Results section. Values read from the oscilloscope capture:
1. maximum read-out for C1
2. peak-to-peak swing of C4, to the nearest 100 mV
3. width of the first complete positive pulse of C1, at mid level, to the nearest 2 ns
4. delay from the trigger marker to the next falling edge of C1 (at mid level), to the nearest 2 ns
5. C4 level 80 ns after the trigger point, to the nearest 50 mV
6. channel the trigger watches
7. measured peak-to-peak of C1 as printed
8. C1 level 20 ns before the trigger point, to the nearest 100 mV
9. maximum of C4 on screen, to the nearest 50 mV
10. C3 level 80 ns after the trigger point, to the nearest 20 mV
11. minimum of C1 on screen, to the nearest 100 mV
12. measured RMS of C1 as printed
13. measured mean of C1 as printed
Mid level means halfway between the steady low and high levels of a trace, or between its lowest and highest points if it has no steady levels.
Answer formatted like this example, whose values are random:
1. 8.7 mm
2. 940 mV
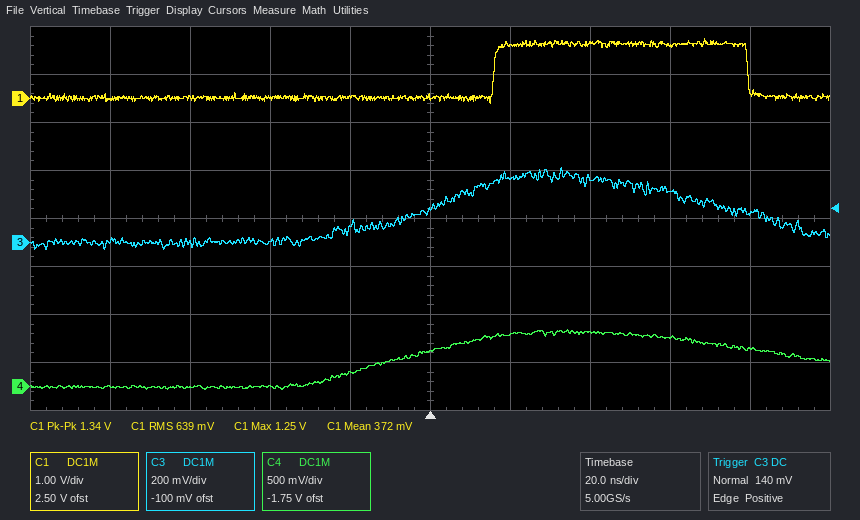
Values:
1. 1.25 V
2. 600 mV
3. 64 ns
4. 80 ns
5. 400 mV
6. C3
7. 1.34 V
8. 0.0 V
9. 600 mV
10. 120 mV
11. -100 mV
12. 639 mV
13. 372 mV
